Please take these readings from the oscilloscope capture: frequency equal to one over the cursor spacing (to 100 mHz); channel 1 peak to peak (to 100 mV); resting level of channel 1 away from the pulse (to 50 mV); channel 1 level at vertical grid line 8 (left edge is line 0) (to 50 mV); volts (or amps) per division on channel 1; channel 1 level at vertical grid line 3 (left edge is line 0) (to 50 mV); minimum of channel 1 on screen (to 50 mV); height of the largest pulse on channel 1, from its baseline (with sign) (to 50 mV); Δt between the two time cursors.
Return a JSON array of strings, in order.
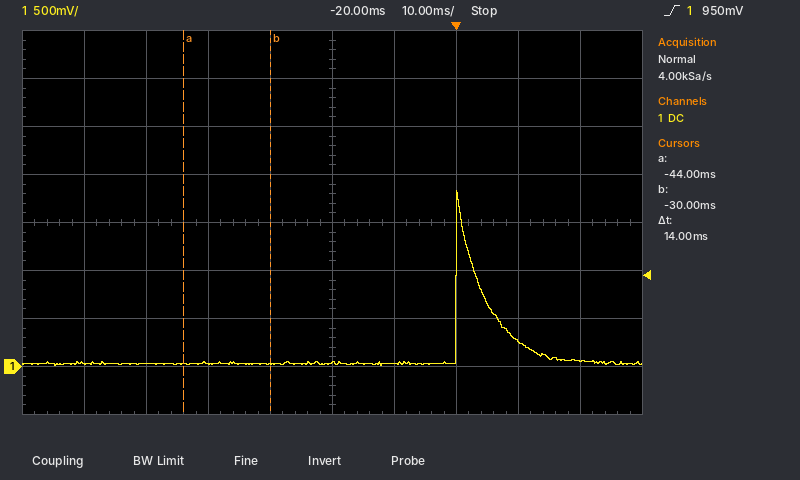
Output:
["71.4 Hz", "1.80 V", "50 mV", "250 mV", "500 mV", "50 mV", "0 mV", "+1.80 V", "14 ms"]
